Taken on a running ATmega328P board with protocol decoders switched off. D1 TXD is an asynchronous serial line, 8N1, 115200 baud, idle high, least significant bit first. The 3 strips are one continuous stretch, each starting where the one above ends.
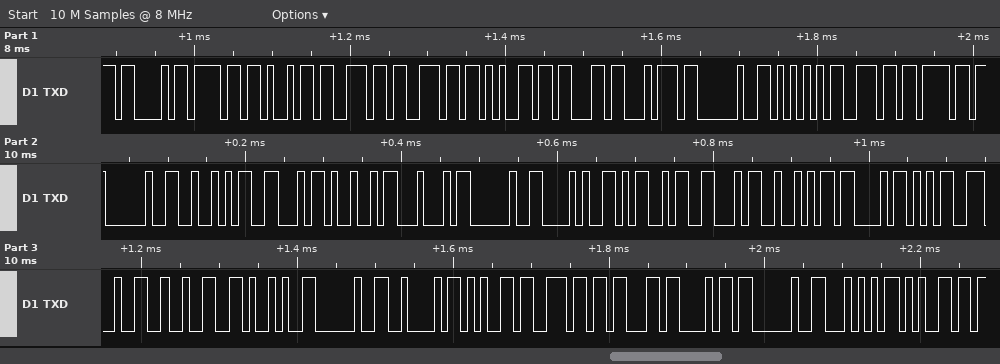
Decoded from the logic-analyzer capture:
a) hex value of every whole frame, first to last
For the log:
43 6F 69 6E 6E 65 63 74 20 55 6E 6F 20 52 46 49 44 20 28 4D 46 52 43 35 32 32 29 20 42 65 6E 63 68 20 54 65
